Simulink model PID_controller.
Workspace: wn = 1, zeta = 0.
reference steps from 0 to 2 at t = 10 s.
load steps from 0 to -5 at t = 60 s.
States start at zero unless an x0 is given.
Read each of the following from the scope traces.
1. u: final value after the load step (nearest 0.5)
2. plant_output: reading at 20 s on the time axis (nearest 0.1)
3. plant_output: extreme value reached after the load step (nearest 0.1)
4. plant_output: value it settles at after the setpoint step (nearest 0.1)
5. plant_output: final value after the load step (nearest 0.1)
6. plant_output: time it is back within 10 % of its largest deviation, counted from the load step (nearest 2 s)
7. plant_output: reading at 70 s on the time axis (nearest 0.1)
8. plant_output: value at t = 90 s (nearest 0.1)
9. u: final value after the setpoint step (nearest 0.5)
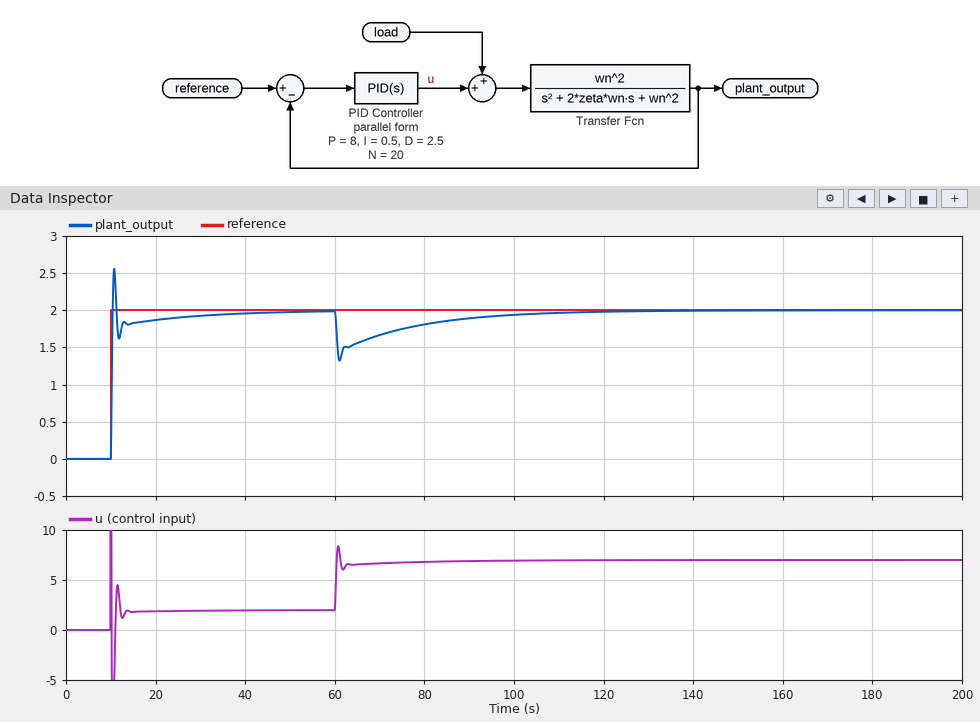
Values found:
7.0
1.9
1.3
2.0
2.0
38 s
1.7
1.9
2.0
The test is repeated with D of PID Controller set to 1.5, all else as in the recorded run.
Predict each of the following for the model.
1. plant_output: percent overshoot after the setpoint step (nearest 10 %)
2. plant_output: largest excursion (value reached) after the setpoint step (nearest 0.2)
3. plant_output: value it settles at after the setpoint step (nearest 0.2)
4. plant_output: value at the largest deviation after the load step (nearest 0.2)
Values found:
40 %
2.8
2.0
1.2
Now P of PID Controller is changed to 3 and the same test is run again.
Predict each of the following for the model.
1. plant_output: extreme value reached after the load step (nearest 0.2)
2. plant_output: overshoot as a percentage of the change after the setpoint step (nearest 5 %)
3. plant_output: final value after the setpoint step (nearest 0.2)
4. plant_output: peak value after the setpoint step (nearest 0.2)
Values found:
0.8
10 %
2.0
2.2
